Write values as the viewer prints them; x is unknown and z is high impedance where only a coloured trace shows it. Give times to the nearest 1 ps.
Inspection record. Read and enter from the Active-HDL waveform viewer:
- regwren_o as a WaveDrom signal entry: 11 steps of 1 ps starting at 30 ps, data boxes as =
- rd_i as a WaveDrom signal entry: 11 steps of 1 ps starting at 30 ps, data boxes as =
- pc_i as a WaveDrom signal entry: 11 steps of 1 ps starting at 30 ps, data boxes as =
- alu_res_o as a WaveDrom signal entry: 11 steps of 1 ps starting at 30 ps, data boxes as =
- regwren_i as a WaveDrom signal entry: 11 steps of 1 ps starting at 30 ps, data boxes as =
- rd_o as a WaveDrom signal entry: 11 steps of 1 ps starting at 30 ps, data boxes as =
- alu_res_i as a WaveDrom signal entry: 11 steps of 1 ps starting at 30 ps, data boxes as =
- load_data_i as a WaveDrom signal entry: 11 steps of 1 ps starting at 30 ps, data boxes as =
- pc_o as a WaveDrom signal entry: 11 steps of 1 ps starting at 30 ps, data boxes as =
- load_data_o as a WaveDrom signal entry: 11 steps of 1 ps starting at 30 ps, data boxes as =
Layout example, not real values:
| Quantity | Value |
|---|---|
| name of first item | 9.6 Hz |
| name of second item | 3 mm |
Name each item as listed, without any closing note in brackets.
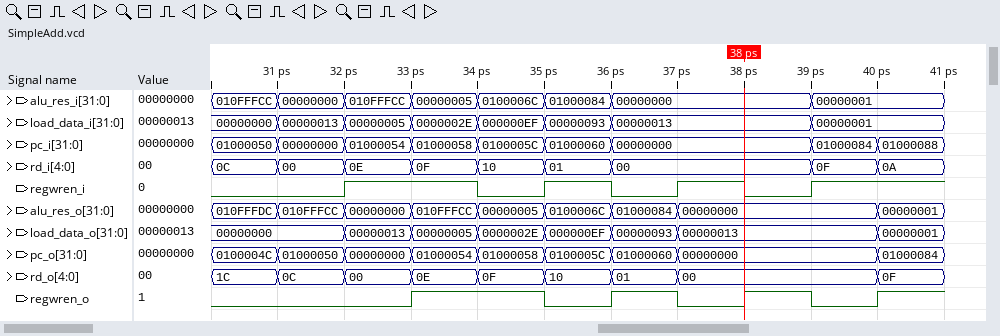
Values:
| Quantity | Value |
|---|---|
| regwren_o as a WaveDrom signal entry: 11 steps of 1 ps starting at 30 ps, data boxes as = | {name: 'regwren_o', wave: '0..1.010101'} |
| rd_i as a WaveDrom signal entry: 11 steps of 1 ps starting at 30 ps, data boxes as = | {name: 'rd_i', wave: '=======..==', data: '0C 00 0E 0F 10 01 00 0F 0A'} |
| pc_i as a WaveDrom signal entry: 11 steps of 1 ps starting at 30 ps, data boxes as = | {name: 'pc_i', wave: '=======..==', data: '01000050 00000000 01000054 01000058 0100005C 01000060 00000000 01000084 01000088'} |
| alu_res_o as a WaveDrom signal entry: 11 steps of 1 ps starting at 30 ps, data boxes as = | {name: 'alu_res_o', wave: '========..=', data: '010FFFDC 010FFFCC 00000000 010FFFCC 00000005 0100006C 01000084 00000000 00000001'} |
| regwren_i as a WaveDrom signal entry: 11 steps of 1 ps starting at 30 ps, data boxes as = | {name: 'regwren_i', wave: '0.1.010101.'} |
| rd_o as a WaveDrom signal entry: 11 steps of 1 ps starting at 30 ps, data boxes as = | {name: 'rd_o', wave: '========..=', data: '1C 0C 00 0E 0F 10 01 00 0F'} |
| alu_res_i as a WaveDrom signal entry: 11 steps of 1 ps starting at 30 ps, data boxes as = | {name: 'alu_res_i', wave: '=======..=.', data: '010FFFCC 00000000 010FFFCC 00000005 0100006C 01000084 00000000 00000001'} |
| load_data_i as a WaveDrom signal entry: 11 steps of 1 ps starting at 30 ps, data boxes as = | {name: 'load_data_i', wave: '=======..=.', data: '00000000 00000013 00000005 0000002E 000000EF 00000093 00000013 00000001'} |
| pc_o as a WaveDrom signal entry: 11 steps of 1 ps starting at 30 ps, data boxes as = | {name: 'pc_o', wave: '========..=', data: '0100004C 01000050 00000000 01000054 01000058 0100005C 01000060 00000000 01000084'} |
| load_data_o as a WaveDrom signal entry: 11 steps of 1 ps starting at 30 ps, data boxes as = | {name: 'load_data_o', wave: '=.======..=', data: '00000000 00000013 00000005 0000002E 000000EF 00000093 00000013 00000001'} |
